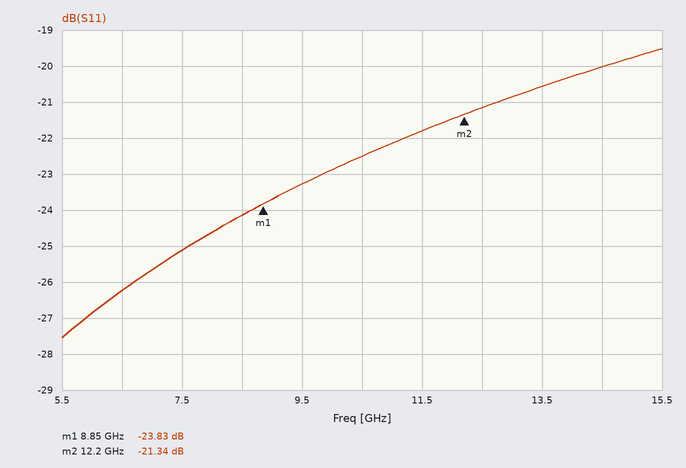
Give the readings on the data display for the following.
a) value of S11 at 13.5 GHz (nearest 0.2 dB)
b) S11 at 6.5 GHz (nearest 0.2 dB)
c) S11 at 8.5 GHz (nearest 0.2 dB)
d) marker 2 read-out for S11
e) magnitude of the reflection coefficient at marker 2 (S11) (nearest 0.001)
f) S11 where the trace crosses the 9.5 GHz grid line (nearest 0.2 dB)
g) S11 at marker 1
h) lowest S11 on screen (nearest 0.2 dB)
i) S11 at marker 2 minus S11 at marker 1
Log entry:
-20.6 dB
-26.2 dB
-24.2 dB
-21.34 dB
0.086
-23.2 dB
-23.83 dB
-27.6 dB
2.49 dB
